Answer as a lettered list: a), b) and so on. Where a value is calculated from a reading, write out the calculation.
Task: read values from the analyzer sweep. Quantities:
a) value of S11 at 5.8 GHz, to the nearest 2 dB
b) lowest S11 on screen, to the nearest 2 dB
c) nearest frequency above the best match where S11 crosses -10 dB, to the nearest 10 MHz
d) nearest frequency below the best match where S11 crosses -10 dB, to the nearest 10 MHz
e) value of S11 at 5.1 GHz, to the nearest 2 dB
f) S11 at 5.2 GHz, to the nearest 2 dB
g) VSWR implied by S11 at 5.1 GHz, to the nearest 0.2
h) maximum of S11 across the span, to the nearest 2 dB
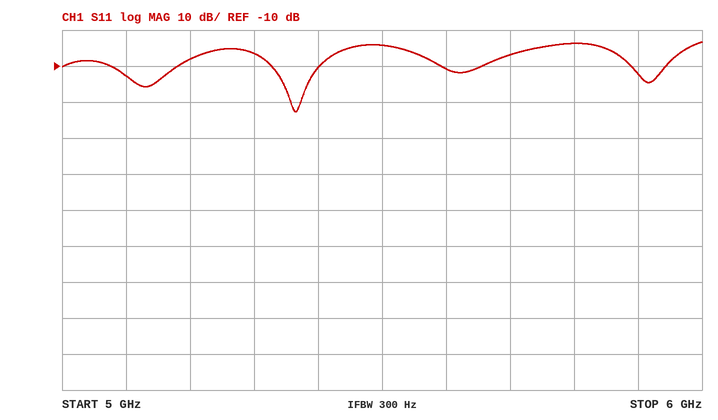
a) -4 dB
b) -22 dB
c) 5.40 GHz
d) 5.33 GHz
e) -12 dB
f) -8 dB
g) |Γ| = 10^(-12/20) = 0.2512; VSWR = (1 + 0.2512)/(1 − 0.2512) ≈ 1.67, so 1.6 to the nearest 0.2
h) -4 dB
